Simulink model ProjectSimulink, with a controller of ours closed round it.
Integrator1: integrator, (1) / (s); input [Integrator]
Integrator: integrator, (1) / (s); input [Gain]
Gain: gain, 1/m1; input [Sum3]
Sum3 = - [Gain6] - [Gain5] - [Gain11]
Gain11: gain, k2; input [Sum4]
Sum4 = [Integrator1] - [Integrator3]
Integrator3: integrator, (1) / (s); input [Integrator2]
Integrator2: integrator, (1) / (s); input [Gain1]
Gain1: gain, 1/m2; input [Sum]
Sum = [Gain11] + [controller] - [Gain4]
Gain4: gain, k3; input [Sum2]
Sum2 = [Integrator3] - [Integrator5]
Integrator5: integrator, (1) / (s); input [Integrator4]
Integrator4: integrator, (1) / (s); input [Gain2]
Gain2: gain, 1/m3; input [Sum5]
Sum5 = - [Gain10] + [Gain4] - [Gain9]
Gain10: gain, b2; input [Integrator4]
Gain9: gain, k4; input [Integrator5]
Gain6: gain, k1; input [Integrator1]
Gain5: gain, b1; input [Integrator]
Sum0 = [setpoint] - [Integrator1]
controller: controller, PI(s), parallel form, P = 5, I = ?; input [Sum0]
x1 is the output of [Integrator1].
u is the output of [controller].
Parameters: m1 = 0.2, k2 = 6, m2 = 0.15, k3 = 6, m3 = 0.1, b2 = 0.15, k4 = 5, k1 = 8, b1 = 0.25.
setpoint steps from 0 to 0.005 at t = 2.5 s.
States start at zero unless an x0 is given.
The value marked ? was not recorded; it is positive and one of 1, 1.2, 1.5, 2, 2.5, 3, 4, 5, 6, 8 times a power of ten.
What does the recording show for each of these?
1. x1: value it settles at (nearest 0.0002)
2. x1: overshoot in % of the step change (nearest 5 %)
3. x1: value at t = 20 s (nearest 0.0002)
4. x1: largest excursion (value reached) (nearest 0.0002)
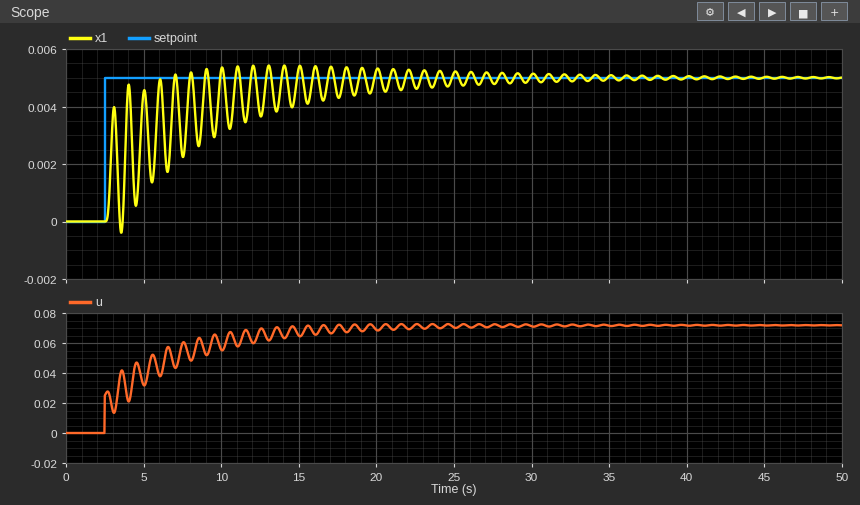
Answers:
0.0050
10 %
0.0052
0.0054
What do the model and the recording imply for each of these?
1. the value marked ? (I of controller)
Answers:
4
